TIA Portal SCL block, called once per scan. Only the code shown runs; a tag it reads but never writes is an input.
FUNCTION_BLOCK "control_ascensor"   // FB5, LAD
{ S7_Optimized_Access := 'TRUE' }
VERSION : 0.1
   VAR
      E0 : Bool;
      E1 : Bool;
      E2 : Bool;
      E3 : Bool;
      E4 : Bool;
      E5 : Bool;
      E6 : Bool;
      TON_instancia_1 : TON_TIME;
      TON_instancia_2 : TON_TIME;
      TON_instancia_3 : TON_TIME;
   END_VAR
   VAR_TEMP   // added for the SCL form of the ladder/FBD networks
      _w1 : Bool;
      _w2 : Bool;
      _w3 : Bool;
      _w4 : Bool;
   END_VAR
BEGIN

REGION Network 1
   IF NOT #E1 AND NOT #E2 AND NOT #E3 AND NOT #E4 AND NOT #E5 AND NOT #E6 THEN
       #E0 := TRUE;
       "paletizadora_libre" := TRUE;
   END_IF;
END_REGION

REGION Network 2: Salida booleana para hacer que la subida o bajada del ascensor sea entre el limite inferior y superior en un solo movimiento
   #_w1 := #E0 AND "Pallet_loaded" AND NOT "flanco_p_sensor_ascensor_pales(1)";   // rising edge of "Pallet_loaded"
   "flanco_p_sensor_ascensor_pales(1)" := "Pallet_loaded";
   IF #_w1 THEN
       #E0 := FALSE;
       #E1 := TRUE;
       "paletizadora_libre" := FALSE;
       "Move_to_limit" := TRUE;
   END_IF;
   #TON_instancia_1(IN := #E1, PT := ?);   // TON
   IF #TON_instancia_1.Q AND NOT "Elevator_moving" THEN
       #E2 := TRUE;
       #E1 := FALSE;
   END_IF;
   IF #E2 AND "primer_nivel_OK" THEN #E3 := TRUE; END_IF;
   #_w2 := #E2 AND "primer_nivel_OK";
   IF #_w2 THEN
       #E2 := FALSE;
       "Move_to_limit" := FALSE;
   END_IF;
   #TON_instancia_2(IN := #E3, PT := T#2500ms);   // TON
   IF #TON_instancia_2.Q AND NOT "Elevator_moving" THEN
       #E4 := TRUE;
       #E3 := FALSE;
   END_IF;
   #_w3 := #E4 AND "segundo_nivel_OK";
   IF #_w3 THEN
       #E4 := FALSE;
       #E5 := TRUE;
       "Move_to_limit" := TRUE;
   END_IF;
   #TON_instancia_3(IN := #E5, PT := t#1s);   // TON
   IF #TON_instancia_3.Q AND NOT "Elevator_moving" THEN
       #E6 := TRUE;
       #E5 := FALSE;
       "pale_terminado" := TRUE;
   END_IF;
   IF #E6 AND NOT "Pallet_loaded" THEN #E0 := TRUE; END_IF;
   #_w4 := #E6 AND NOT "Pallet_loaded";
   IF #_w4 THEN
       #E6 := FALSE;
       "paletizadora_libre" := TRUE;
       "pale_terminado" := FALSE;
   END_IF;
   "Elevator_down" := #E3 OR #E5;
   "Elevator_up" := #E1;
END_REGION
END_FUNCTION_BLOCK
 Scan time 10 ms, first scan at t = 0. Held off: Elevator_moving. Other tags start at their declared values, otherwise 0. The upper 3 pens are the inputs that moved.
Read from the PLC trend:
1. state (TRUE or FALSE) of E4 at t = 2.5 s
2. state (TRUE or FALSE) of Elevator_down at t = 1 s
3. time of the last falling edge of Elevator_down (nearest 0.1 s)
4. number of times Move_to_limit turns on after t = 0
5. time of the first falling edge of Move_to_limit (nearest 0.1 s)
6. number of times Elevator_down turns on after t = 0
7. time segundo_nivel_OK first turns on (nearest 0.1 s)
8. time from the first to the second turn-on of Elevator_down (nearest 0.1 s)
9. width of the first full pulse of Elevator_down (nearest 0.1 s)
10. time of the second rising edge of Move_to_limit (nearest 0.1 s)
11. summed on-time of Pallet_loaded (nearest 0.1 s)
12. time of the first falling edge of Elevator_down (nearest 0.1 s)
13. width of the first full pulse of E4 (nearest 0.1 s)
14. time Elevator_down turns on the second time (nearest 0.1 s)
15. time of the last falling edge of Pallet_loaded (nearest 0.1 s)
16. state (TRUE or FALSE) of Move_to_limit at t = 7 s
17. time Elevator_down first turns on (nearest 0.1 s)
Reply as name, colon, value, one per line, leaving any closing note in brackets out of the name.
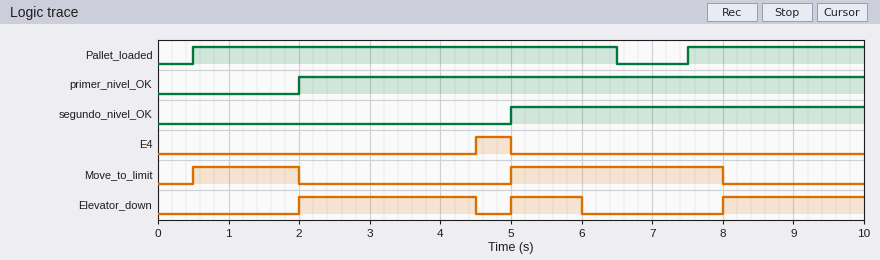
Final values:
state (TRUE or FALSE) of E4 at t = 2.5 s: FALSE
state (TRUE or FALSE) of Elevator_down at t = 1 s: FALSE
time of the last falling edge of Elevator_down: 6.0 s
number of times Move_to_limit turns on after t = 0: 2
time of the first falling edge of Move_to_limit: 2.0 s
number of times Elevator_down turns on after t = 0: 3
time segundo_nivel_OK first turns on: 5.0 s
time from the first to the second turn-on of Elevator_down: 3.0 s
width of the first full pulse of Elevator_down: 2.5 s
time of the second rising edge of Move_to_limit: 5.0 s
summed on-time of Pallet_loaded: 8.5 s
time of the first falling edge of Elevator_down: 4.5 s
width of the first full pulse of E4: 0.5 s
time Elevator_down turns on the second time: 5.0 s
time of the last falling edge of Pallet_loaded: 6.5 s
state (TRUE or FALSE) of Move_to_limit at t = 7 s: TRUE
time Elevator_down first turns on: 2.0 s
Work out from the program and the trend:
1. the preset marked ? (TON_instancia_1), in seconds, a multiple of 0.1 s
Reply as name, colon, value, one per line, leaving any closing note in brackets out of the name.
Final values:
the preset marked ? (TON_instancia_1), in seconds, a multiple of 0.1 s: 0.5 s
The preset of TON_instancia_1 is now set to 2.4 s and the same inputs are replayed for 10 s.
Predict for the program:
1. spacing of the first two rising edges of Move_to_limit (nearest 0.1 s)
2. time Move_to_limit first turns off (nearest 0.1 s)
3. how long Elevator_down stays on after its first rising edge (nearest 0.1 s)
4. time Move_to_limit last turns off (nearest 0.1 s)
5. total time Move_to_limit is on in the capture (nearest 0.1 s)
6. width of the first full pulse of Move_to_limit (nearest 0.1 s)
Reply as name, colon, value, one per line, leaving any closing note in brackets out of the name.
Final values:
spacing of the first two rising edges of Move_to_limit: 4.9 s
time Move_to_limit first turns off: 2.9 s
how long Elevator_down stays on after its first rising edge: 3.5 s
time Move_to_limit last turns off: 9.9 s
total time Move_to_limit is on in the capture: 6.9 s
width of the first full pulse of Move_to_limit: 2.4 s
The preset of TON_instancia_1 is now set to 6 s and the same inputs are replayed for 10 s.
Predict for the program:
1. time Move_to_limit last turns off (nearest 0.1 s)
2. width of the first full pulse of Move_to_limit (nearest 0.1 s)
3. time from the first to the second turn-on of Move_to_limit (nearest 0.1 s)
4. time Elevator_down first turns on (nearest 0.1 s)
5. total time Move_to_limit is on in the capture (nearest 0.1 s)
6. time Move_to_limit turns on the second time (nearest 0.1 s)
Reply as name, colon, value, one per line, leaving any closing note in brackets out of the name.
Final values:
time Move_to_limit last turns off: 6.5 s
width of the first full pulse of Move_to_limit: 6.0 s
time from the first to the second turn-on of Move_to_limit: 8.5 s
time Elevator_down first turns on: 6.5 s
total time Move_to_limit is on in the capture: 7.0 s
time Move_to_limit turns on the second time: 9.0 s
